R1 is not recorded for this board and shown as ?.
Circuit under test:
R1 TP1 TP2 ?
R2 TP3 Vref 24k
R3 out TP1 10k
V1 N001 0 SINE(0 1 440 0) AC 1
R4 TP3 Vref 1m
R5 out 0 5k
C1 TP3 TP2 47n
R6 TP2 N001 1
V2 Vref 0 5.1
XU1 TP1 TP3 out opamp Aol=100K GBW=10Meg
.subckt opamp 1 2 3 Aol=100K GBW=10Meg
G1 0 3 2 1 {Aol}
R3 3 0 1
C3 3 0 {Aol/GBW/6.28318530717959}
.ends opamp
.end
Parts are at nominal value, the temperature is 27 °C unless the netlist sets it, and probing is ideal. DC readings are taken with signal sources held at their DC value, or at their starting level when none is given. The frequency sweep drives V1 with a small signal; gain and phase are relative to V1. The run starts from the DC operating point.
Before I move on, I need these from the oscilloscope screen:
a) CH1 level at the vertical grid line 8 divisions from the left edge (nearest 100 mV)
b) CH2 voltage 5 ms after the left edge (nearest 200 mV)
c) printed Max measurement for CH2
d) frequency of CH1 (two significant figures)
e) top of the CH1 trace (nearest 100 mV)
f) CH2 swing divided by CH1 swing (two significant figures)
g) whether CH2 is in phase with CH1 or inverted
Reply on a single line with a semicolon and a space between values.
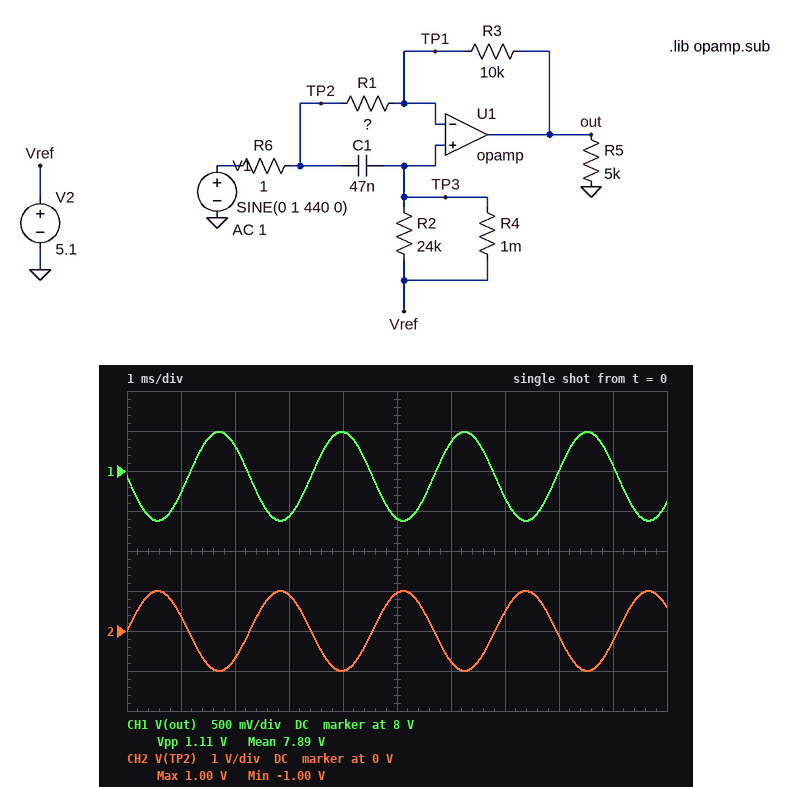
8.0 V; 1.0 V; 1.00 V; 440 Hz; 8.5 V; 1.8; inverted
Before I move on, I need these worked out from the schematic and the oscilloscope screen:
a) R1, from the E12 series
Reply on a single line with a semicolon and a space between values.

18 kΩ
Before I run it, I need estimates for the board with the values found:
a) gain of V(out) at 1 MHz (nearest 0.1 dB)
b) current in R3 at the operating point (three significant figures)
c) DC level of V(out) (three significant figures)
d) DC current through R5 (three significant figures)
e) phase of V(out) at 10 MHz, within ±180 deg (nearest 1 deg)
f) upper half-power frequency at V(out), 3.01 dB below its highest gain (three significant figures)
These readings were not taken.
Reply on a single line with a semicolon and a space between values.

-5.6 dB; 283 µA; 7.93 V; 1.59 mA; 51 deg; 2.79 MHz
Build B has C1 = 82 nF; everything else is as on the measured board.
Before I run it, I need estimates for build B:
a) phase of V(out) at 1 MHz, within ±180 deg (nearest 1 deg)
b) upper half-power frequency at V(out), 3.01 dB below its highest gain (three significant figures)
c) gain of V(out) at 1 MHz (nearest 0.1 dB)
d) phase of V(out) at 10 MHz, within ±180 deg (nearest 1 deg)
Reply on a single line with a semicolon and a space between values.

144 deg; 1.79 MHz; -6.2 dB; 43 deg
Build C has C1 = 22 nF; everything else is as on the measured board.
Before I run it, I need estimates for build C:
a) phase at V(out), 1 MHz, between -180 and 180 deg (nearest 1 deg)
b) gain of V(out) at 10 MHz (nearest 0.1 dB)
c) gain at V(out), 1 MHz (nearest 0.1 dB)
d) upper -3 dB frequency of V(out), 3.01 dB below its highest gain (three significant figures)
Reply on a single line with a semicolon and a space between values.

163 deg; -15.1 dB; -5.3 dB; 4.38 MHz
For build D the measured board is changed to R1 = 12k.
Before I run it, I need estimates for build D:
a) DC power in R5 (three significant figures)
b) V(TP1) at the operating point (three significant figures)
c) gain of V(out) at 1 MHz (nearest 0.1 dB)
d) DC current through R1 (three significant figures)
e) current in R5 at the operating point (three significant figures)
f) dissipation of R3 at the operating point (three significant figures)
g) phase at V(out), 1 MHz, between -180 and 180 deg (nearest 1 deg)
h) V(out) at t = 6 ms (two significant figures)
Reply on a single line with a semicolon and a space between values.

17.5 mW; 5.10 V; -2.1 dB; 425 µA; 1.87 mA; 1.81 mW; 153 deg; 10 V
